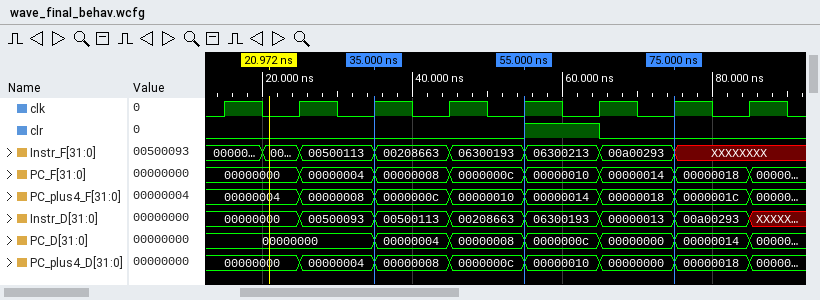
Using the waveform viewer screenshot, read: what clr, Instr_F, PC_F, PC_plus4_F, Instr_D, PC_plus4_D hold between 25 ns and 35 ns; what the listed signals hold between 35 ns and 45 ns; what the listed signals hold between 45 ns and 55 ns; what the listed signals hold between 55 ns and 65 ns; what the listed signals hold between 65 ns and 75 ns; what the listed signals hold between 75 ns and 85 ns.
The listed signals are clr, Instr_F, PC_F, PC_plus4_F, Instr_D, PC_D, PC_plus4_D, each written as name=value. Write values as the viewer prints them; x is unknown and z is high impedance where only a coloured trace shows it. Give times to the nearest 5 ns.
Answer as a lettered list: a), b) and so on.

a) clr=0, Instr_F=00500113, PC_F=00000004, PC_plus4_F=00000008, Instr_D=00500093, PC_plus4_D=00000004
b) clr=0, Instr_F=00208663, PC_F=00000008, PC_plus4_F=0000000c, Instr_D=00500113, PC_D=00000004, PC_plus4_D=00000008
c) clr=0, Instr_F=06300193, PC_F=0000000c, PC_plus4_F=00000010, Instr_D=00208663, PC_D=00000008, PC_plus4_D=0000000c
d) clr=1, Instr_F=06300213, PC_F=00000010, PC_plus4_F=00000014, Instr_D=06300193, PC_D=0000000c, PC_plus4_D=00000010
e) clr=0, Instr_F=00a00293, PC_F=00000014, PC_plus4_F=00000018, Instr_D=00000013, PC_D=00000000, PC_plus4_D=00000000
f) clr=0, Instr_F=XXXXXXXX, PC_F=00000018, PC_plus4_F=0000001c, Instr_D=00a00293, PC_D=00000014, PC_plus4_D=00000018
